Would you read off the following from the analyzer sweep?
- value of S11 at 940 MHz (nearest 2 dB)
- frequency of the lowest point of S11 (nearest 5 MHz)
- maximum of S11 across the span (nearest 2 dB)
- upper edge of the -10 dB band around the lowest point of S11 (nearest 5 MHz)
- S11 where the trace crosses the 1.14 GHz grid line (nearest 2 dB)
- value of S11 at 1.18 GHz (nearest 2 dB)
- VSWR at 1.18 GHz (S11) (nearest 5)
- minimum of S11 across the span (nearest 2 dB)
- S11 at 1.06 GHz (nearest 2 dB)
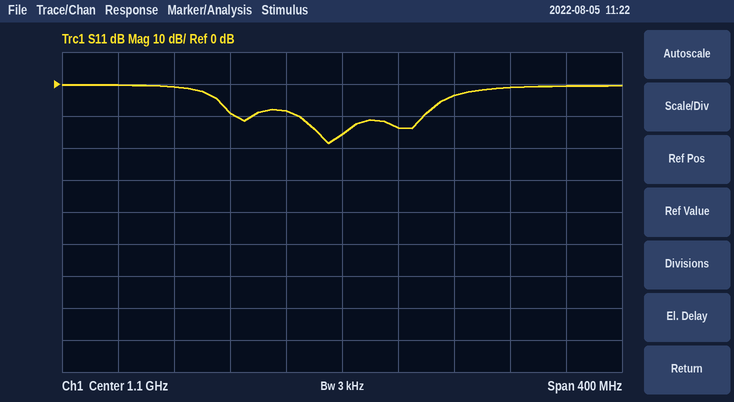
0 dB
1.090 GHz
0 dB
1.160 GHz
-14 dB
-4 dB
5
-18 dB
-8 dB
